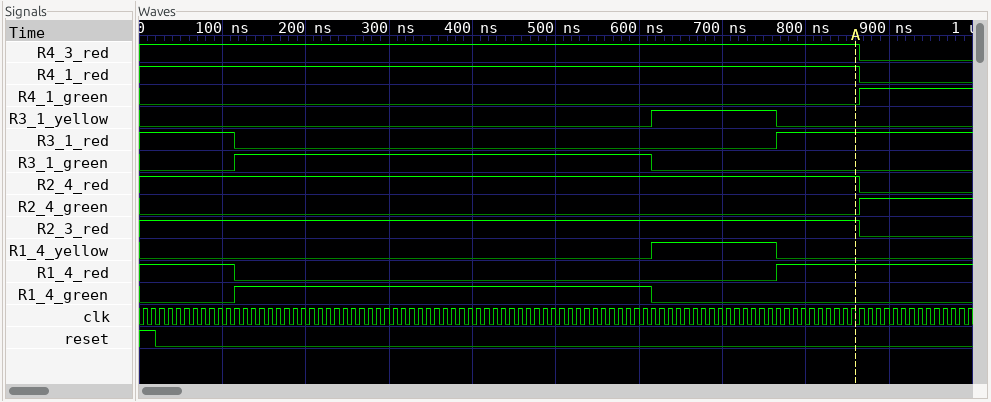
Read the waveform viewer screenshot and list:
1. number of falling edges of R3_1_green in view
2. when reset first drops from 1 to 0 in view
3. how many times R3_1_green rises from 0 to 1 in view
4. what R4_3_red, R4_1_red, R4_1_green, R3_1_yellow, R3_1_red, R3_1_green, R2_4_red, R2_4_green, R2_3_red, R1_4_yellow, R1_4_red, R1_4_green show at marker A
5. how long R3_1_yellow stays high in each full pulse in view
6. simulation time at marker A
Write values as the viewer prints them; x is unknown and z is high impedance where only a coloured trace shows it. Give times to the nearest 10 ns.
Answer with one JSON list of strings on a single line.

["1", "20 ns", "1", "R4_3_red=1, R4_1_red=1, R4_1_green=0, R3_1_yellow=0, R3_1_red=1, R3_1_green=0, R2_4_red=1, R2_4_green=0, R2_3_red=1, R1_4_yellow=0, R1_4_red=1, R1_4_green=0", "150 ns", "860 ns"]
